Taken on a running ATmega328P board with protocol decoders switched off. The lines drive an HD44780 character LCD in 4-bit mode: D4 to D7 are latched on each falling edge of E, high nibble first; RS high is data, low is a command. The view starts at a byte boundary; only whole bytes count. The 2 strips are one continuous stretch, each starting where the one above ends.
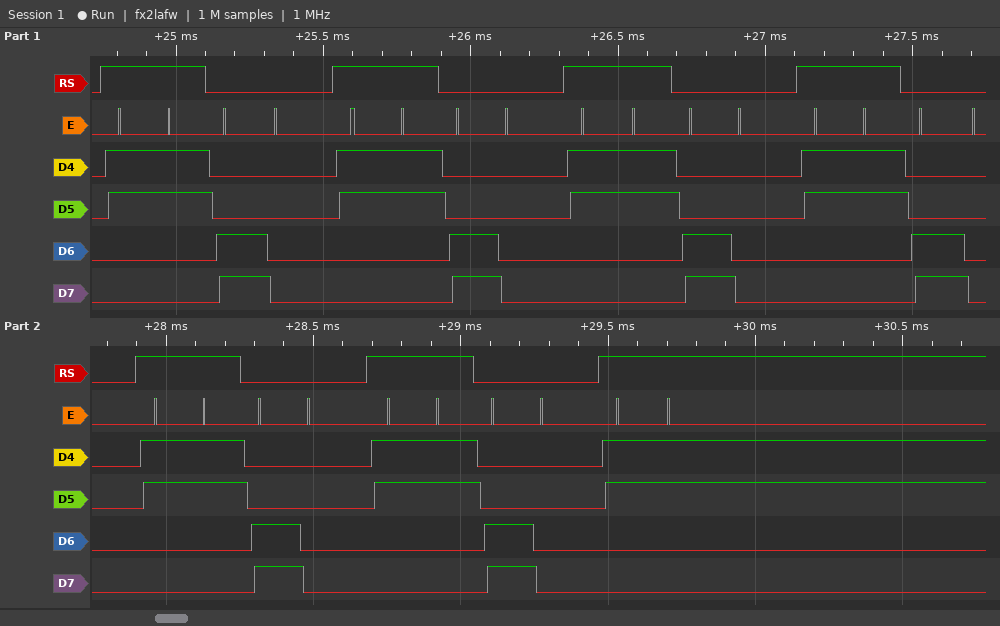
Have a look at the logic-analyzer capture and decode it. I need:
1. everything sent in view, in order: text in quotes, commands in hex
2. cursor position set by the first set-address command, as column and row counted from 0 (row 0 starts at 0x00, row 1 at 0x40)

"3" 0xC0 "3" 0xC0 "3" 0xC0 "3" 0xC0 "3" 0xC0 "3" 0xC0 "3"
column 0, row 1
